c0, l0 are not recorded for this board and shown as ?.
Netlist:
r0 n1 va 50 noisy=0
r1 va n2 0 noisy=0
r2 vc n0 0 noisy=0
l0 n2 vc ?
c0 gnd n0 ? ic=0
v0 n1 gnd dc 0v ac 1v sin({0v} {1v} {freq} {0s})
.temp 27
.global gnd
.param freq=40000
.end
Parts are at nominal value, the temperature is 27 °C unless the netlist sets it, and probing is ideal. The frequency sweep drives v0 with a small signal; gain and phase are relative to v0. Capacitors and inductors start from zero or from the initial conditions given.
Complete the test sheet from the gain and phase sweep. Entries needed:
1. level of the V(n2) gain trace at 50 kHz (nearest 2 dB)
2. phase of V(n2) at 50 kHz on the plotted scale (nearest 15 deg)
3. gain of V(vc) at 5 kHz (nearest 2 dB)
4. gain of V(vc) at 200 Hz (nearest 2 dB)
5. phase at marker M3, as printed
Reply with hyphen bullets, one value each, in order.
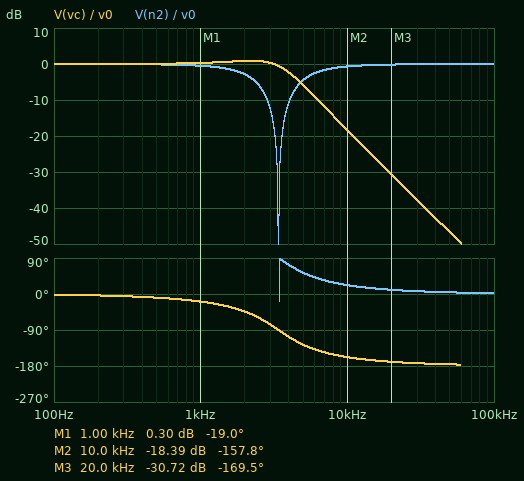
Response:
- 0 dB
- 0 deg
- -6 dB
- 0 dB
- -169.5 deg
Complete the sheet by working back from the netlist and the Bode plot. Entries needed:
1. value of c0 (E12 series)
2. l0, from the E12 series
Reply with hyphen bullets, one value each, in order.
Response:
- 1 µF
- 2.2 mH
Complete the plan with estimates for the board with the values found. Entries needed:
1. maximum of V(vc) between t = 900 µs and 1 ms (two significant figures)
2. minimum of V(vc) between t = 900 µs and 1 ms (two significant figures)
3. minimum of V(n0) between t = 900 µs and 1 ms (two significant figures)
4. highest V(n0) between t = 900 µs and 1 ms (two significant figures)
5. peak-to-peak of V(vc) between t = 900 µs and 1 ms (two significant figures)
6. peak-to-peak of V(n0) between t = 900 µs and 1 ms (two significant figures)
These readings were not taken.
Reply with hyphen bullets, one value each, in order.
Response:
- 7.2 mV
- -7.2 mV
- -7.2 mV
- 7.2 mV
- 14 mV
- 14 mV
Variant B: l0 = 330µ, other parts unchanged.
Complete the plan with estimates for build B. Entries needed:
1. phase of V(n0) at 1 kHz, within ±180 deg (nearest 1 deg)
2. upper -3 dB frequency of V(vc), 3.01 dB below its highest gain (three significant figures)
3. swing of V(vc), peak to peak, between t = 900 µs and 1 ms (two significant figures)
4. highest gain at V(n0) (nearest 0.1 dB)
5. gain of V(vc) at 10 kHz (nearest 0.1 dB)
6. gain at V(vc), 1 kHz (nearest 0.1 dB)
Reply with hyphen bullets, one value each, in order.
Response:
- -18 deg
- 3.66 kHz
- 85 mV
- 0 dB
- -10.0 dB
- -0.3 dB
